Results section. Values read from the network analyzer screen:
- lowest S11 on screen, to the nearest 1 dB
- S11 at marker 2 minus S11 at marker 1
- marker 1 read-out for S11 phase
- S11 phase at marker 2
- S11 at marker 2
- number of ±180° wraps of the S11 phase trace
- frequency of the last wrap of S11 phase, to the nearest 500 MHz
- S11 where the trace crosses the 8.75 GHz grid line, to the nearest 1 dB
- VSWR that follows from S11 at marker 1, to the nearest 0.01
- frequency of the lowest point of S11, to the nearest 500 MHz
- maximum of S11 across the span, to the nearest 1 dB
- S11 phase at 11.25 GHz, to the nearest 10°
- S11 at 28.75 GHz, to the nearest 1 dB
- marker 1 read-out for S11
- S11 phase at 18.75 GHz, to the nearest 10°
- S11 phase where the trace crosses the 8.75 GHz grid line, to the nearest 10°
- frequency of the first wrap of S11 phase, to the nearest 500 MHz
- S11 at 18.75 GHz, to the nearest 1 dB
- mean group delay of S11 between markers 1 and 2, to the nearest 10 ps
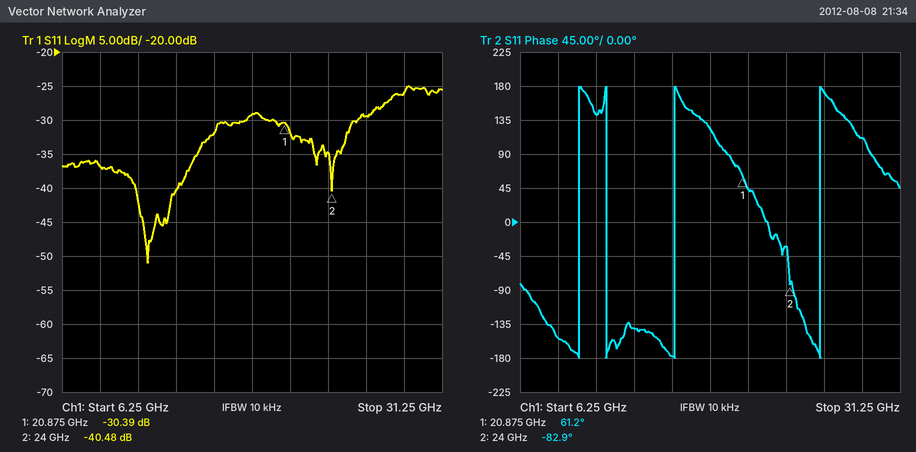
-51 dB
-10.09 dB
61.2°
-82.9°
-40.48 dB
4
26.0 GHz
-37 dB
1.06
12.0 GHz
-25 dB
140°
-26 dB
-30.39 dB
120°
-150°
10.0 GHz
-29 dB
130 ps
